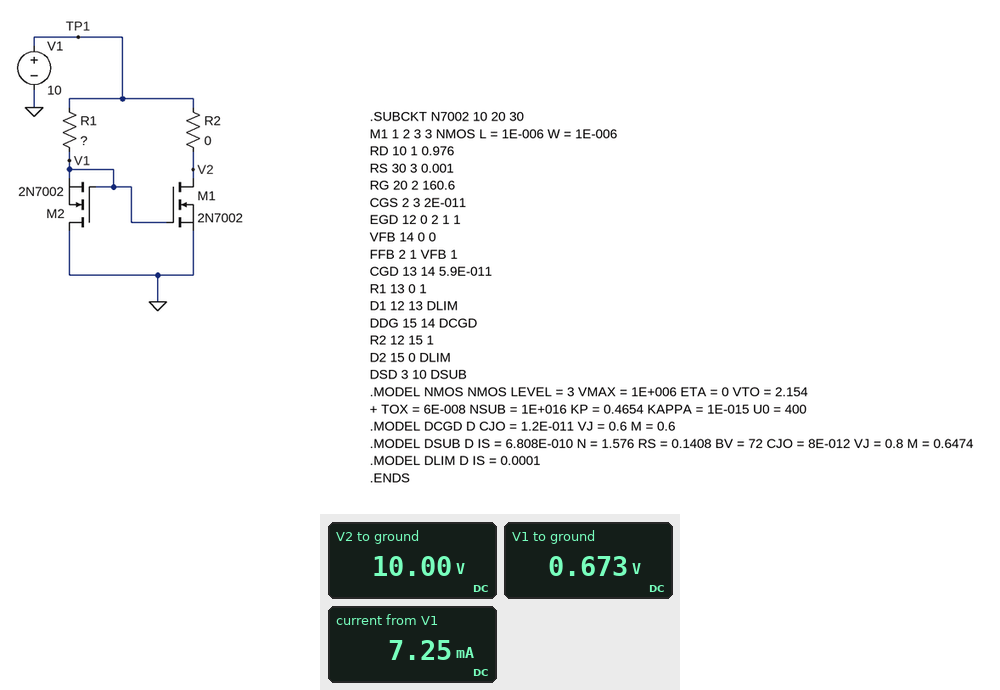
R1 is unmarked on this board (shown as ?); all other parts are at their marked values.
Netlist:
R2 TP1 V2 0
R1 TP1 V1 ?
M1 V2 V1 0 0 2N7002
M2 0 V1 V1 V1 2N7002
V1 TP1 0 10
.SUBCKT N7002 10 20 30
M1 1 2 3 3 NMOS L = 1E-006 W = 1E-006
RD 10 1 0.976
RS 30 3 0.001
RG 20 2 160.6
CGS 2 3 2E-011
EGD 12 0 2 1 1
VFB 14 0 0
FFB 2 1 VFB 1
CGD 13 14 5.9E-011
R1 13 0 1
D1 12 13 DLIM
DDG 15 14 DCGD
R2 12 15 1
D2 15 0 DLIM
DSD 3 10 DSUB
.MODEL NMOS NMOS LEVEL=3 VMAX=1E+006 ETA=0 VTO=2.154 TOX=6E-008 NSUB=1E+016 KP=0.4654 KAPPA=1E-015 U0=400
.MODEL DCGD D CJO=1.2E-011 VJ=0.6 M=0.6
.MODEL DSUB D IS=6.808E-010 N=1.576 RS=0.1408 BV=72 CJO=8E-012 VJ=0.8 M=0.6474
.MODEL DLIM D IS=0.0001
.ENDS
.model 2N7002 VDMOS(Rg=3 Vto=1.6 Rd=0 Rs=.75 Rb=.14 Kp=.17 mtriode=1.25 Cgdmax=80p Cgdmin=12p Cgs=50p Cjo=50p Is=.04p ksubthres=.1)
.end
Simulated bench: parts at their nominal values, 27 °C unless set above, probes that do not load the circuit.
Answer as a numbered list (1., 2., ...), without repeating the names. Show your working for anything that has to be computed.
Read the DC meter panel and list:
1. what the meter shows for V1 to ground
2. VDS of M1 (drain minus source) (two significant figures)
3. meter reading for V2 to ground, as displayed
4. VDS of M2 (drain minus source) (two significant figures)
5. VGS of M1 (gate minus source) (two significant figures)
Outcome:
1. 0.673 V
2. 10 V = 10 V
3. 10.00 V
4. 0 V - 673 mV = -670 mV
5. 673 mV = 670 mV
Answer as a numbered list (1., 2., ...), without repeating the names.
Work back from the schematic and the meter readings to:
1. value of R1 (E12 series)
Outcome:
1. 1.2 kΩ
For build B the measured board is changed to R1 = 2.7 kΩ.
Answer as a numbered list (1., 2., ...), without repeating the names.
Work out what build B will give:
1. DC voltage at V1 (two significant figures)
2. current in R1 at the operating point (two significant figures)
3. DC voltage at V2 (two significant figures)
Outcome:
1. 650 mV
2. 3.5 mA
3. 10 V
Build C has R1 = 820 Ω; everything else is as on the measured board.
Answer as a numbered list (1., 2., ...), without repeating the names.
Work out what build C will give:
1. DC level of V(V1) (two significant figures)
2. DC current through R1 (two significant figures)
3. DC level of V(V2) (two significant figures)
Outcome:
1. 680 mV
2. 11 mA
3. 10 V
